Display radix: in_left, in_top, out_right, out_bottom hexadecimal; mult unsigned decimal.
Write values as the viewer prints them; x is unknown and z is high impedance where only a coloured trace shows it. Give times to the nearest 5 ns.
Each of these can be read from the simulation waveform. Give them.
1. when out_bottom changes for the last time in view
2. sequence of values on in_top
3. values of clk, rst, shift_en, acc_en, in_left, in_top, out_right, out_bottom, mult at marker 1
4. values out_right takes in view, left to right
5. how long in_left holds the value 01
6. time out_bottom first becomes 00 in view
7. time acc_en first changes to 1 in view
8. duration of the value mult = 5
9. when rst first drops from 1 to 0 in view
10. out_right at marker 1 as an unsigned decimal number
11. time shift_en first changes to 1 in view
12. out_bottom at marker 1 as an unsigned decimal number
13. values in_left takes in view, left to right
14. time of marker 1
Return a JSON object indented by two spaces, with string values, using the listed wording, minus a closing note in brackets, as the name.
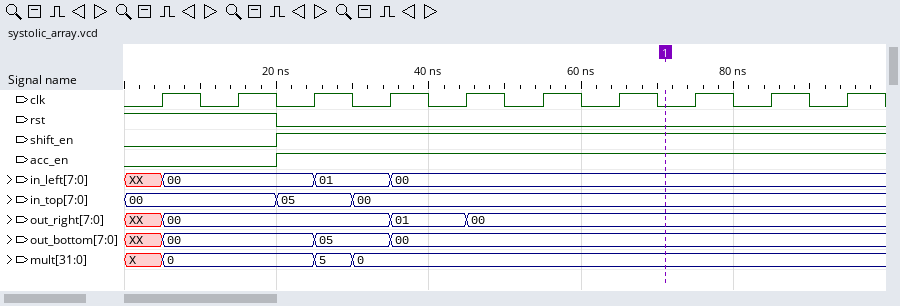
{
  "when out_bottom changes for the last time in view": "35 ns",
  "sequence of values on in_top": "00, 05, 00",
  "values of clk, rst, shift_en, acc_en, in_left, in_top, out_right, out_bottom, mult at marker 1": "clk=0, rst=0, shift_en=1, acc_en=1, in_left=00, in_top=00, out_right=00, out_bottom=00, mult=0",
  "values out_right takes in view, left to right": "XX, 00, 01, 00",
  "how long in_left holds the value 01": "10 ns",
  "time out_bottom first becomes 00 in view": "5 ns",
  "time acc_en first changes to 1 in view": "20 ns",
  "duration of the value mult = 5": "5 ns",
  "when rst first drops from 1 to 0 in view": "20 ns",
  "out_right at marker 1 as an unsigned decimal number": "0",
  "time shift_en first changes to 1 in view": "20 ns",
  "out_bottom at marker 1 as an unsigned decimal number": "0",
  "values in_left takes in view, left to right": "XX, 00, 01, 00",
  "time of marker 1": "70 ns"
}
